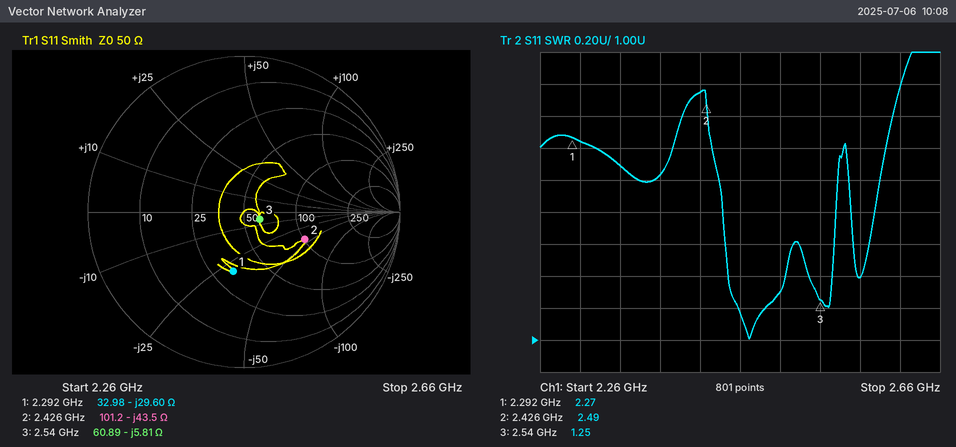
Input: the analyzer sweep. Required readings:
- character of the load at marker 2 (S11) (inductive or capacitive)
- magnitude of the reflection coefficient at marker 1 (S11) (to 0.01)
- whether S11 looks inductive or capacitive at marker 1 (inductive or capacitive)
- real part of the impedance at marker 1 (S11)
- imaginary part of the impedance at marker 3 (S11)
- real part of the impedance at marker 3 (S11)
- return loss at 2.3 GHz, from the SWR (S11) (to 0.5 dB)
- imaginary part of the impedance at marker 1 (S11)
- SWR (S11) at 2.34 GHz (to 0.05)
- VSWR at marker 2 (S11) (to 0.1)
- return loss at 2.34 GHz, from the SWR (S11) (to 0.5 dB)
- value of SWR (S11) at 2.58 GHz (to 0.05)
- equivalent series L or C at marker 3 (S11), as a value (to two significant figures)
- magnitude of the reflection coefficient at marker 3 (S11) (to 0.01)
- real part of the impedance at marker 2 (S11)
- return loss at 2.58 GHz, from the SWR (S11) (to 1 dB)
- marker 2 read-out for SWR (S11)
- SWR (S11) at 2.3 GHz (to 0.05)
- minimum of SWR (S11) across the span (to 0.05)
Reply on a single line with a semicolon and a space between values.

capacitive; 0.39; capacitive; 32.98 Ω; -5.81 Ω; 60.89 Ω; 8.5 dB; -29.60 Ω; 2.10; 2.5; 9.0 dB; 1.40; 11 pF; 0.11; 101.2 Ω; 16 dB; 2.49; 2.25; 1.00
